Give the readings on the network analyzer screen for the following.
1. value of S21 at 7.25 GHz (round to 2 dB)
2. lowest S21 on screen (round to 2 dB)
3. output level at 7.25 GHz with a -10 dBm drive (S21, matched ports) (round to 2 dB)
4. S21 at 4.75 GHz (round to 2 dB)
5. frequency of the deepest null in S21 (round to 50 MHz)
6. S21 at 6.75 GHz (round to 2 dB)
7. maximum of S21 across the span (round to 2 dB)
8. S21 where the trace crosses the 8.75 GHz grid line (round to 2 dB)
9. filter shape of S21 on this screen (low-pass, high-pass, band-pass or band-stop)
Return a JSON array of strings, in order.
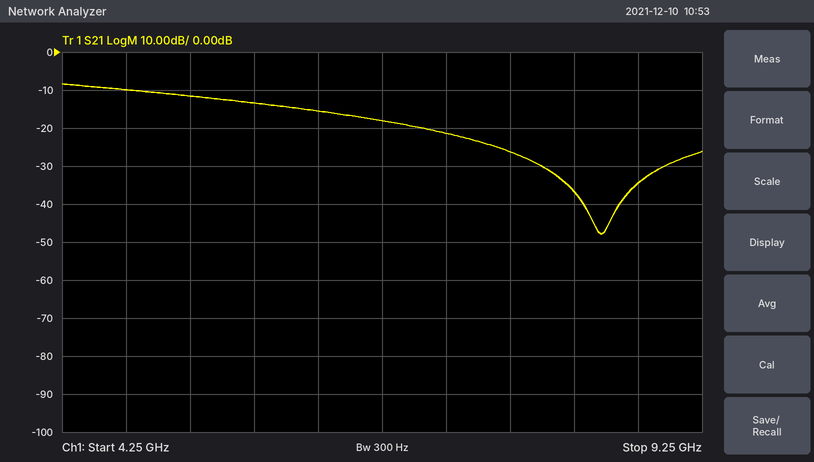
["-22 dB", "-48 dB", "-32 dBm", "-10 dB", "8.45 GHz", "-18 dB", "-8 dB", "-34 dB", "low-pass"]
